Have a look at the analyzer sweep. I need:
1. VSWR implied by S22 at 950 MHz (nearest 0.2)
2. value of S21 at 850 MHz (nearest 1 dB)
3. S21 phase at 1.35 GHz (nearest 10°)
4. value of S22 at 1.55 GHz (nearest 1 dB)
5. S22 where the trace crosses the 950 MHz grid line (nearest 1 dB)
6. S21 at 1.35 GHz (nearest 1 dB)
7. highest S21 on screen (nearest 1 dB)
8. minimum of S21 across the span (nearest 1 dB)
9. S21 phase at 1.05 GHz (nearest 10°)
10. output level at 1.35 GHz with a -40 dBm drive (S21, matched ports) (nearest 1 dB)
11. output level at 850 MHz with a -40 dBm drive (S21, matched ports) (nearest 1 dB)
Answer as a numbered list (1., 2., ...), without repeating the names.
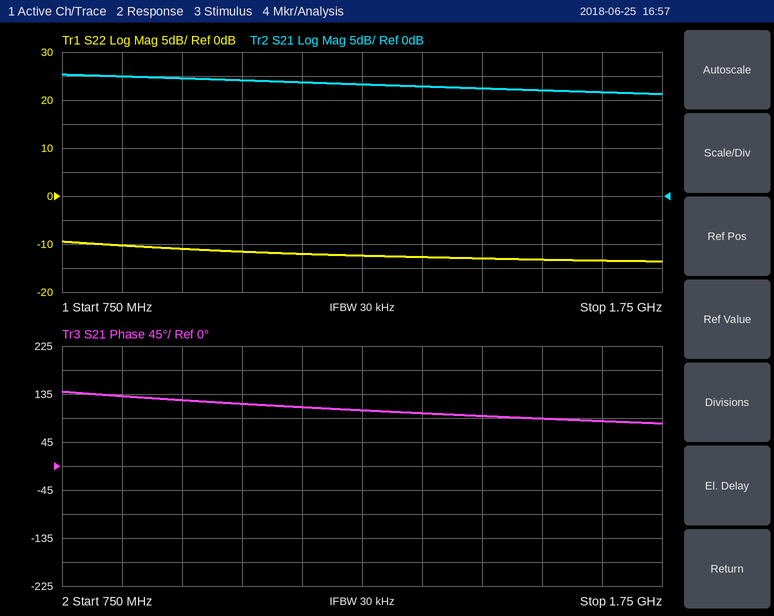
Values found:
1. 1.8
2. 25 dB
3. 100°
4. -13 dB
5. -11 dB
6. 23 dB
7. 25 dB
8. 21 dB
9. 120°
10. -17 dBm
11. -15 dBm
